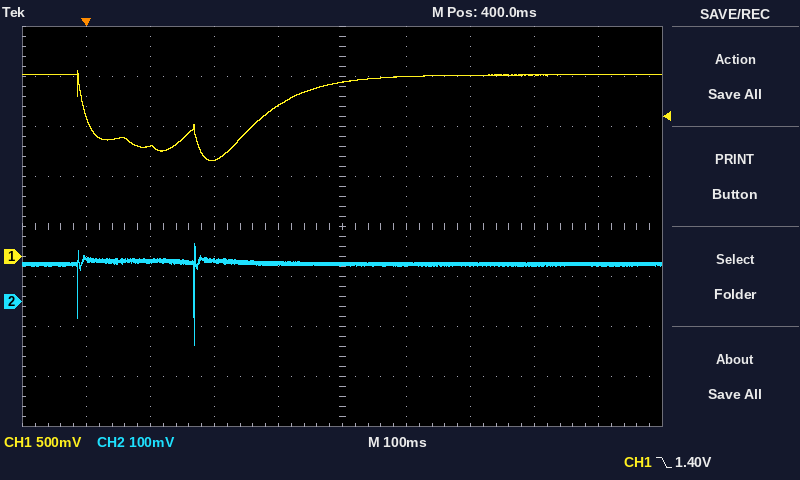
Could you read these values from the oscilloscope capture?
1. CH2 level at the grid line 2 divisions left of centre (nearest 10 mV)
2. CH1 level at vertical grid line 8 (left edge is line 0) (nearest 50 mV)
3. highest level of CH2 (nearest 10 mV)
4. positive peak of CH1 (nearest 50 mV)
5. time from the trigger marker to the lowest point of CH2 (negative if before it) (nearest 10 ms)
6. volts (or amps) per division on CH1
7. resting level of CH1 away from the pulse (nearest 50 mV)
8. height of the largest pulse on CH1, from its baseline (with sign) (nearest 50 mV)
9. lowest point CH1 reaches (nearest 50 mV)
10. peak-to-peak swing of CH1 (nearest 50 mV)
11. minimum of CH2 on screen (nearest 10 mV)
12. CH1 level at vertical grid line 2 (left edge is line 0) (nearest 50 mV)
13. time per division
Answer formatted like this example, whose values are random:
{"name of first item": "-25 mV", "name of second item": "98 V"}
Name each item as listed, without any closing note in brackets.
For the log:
{"CH2 level at the grid line 2 divisions left of centre": "80 mV", "CH1 level at vertical grid line 8 (left edge is line 0)": "1.80 V", "highest level of CH2": "120 mV", "positive peak of CH1": "1.85 V", "time from the trigger marker to the lowest point of CH2 (negative if before it)": "+170 ms", "volts (or amps) per division on CH1": "500 mV", "resting level of CH1 away from the pulse": "1.80 V", "height of the largest pulse on CH1, from its baseline (with sign)": "-850 mV", "lowest point CH1 reaches": "950 mV", "peak-to-peak swing of CH1": "900 mV", "minimum of CH2 on screen": "-90 mV", "CH1 level at vertical grid line 2 (left edge is line 0)": "1.10 V", "time per division": "100 ms"}
